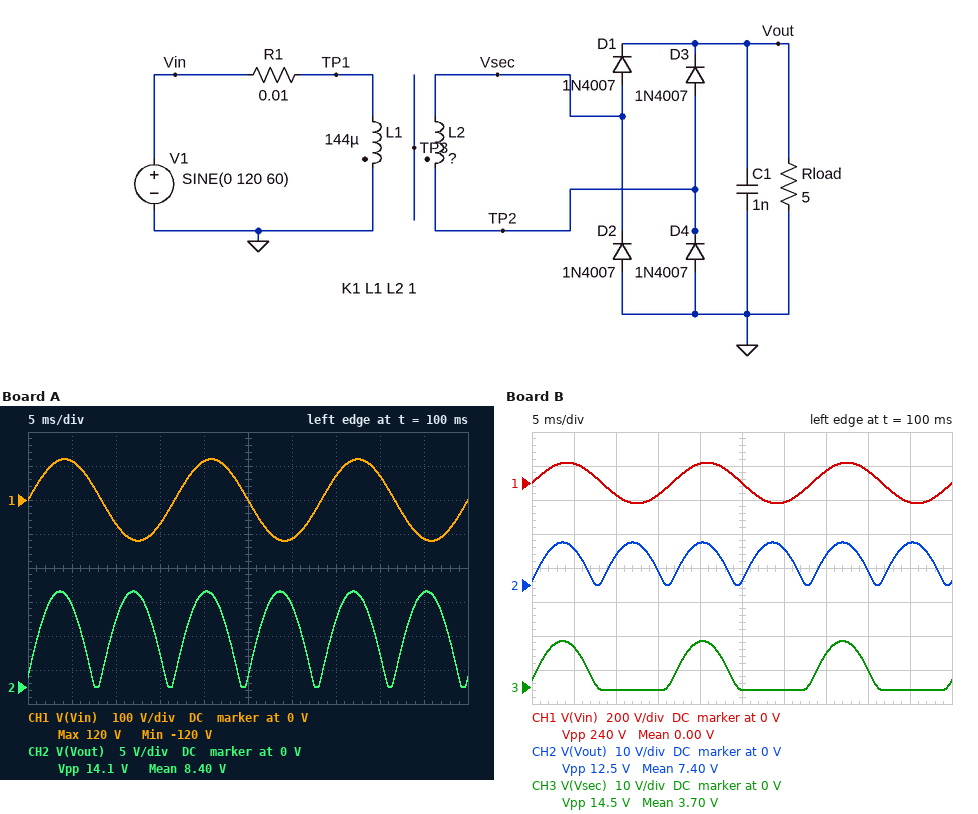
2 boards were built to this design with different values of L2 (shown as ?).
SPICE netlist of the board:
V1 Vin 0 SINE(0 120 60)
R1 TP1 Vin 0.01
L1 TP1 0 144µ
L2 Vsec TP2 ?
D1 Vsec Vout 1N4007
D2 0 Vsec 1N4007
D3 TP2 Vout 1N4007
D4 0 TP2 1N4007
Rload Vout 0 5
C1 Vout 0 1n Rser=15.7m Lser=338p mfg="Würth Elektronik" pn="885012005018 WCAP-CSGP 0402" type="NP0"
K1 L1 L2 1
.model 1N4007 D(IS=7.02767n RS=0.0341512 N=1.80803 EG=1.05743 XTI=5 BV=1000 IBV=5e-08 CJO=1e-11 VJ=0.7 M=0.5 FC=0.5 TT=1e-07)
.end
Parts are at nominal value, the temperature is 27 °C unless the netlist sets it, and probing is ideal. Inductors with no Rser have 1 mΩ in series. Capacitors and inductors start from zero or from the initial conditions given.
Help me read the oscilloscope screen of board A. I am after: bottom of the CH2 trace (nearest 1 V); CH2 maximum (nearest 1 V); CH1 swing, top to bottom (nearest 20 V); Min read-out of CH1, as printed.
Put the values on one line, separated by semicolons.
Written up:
0 V; 14 V; 240 V; -120 V
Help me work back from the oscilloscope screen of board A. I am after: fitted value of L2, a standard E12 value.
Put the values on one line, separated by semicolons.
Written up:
2.7 µH
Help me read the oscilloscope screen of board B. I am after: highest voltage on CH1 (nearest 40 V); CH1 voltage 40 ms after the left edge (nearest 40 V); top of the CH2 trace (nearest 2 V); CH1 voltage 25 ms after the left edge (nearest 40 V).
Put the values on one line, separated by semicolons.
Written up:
120 V; 80 V; 12 V; 0 V
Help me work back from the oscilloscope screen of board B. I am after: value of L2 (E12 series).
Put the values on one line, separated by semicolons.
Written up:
2.2 µH
